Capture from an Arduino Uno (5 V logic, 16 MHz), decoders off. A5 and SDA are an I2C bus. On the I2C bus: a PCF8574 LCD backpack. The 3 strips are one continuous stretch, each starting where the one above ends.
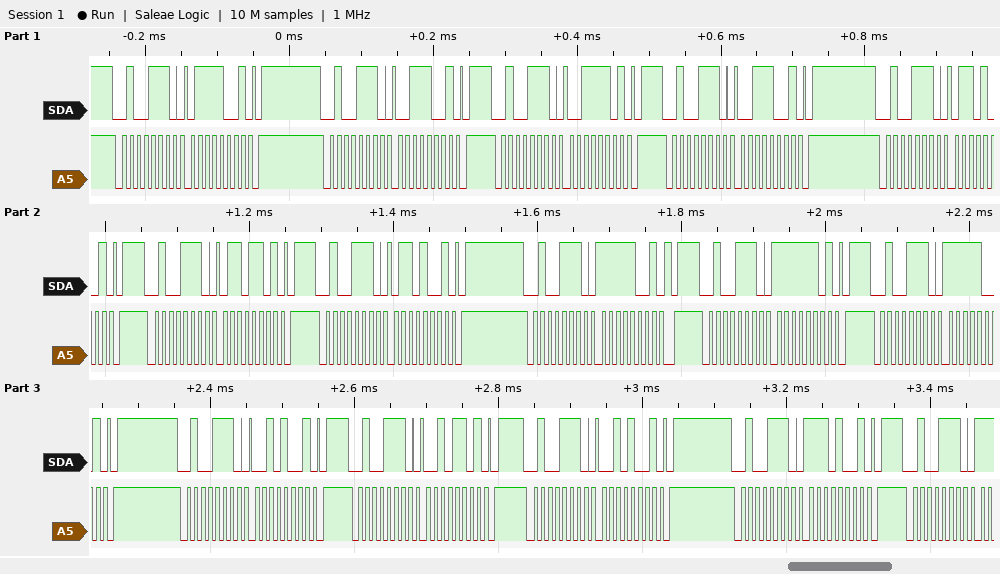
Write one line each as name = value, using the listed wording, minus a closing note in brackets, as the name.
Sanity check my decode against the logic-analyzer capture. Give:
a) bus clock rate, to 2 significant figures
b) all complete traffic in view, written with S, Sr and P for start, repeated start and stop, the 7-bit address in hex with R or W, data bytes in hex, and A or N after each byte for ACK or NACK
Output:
bus clock rate, to 2 significant figures = 100 kHz
all complete traffic in view, written with S, Sr and P for start, repeated start and stop, the 7-bit address in hex with R or W, data bytes in hex, and A or N after each byte for ACK or NACK = S 27W A 79 A P S 27W A 39 A P S 27W A 3D A P S 27W A 39 A P S 27W A 69 A P S 27W A 6D A P S 27W A 69 A P S 27W A F9 A P S 27W A FD A P S 27W A F9 A P S 27W A 29 A P S 27W A 2D A P S 27W A 29 A P S 27W A E9 A P S 27W A
